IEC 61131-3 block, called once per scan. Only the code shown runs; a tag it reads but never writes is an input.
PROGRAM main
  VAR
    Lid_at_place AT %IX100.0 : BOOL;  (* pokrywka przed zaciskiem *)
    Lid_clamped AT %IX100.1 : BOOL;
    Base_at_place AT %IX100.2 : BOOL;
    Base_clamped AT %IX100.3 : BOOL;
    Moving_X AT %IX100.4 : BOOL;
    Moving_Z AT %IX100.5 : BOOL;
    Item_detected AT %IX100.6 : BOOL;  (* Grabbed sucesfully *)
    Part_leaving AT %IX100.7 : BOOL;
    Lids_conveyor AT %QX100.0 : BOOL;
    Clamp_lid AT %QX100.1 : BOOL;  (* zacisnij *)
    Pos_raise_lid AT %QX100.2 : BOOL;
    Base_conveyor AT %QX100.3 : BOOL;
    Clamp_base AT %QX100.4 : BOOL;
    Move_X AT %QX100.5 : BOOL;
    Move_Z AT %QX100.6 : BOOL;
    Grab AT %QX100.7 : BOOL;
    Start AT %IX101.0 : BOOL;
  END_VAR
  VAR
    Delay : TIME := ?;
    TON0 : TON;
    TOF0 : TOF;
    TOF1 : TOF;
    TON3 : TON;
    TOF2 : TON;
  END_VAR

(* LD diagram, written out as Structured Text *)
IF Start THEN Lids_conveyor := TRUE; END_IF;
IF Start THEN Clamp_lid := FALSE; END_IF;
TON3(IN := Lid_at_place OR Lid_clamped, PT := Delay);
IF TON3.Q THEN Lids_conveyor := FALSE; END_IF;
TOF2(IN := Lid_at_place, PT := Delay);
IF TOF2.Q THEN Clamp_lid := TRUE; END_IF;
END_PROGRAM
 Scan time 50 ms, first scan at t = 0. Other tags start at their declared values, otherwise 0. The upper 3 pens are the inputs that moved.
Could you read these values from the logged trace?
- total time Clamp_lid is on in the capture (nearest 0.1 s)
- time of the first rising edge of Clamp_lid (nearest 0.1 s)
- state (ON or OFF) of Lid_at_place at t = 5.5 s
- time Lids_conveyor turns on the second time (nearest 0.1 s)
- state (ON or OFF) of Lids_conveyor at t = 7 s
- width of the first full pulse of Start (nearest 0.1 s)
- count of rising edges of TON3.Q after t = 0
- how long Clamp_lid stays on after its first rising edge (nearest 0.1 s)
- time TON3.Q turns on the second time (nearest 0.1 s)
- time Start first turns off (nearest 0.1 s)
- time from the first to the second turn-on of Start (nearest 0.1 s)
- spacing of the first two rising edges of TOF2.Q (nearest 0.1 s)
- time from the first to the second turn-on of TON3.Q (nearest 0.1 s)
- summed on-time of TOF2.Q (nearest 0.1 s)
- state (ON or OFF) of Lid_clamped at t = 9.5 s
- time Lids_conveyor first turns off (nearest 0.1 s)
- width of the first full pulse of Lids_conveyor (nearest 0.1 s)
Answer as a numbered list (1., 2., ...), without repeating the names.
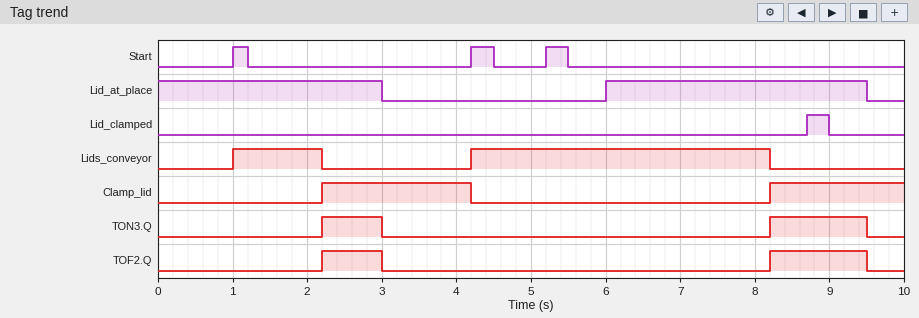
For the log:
1. 3.8 s
2. 2.2 s
3. OFF
4. 4.2 s
5. ON
6. 0.2 s
7. 2
8. 2.0 s
9. 8.2 s
10. 1.2 s
11. 3.2 s
12. 6.0 s
13. 6.0 s
14. 2.1 s
15. OFF
16. 2.2 s
17. 1.2 s
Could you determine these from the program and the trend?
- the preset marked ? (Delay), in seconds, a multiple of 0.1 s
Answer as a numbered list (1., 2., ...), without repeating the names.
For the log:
1. 2.2 s
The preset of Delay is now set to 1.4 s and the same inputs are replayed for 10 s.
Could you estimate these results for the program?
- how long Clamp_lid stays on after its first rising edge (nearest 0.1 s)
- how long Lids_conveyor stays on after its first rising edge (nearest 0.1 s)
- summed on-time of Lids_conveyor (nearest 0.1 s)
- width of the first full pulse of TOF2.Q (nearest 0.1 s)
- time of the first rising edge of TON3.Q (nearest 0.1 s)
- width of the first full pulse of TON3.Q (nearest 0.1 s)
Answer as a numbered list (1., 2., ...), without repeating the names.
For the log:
1. 2.8 s
2. 0.4 s
3. 3.6 s
4. 1.6 s
5. 1.4 s
6. 1.6 s
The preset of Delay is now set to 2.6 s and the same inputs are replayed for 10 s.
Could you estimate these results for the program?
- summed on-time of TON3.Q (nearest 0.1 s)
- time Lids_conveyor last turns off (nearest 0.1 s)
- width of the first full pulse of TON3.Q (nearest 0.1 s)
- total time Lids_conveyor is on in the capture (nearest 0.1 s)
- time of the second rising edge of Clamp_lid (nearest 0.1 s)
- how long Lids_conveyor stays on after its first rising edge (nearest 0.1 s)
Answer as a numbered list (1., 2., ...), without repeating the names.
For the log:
1. 1.3 s
2. 8.6 s
3. 0.4 s
4. 6.0 s
5. 8.6 s
6. 1.6 s
